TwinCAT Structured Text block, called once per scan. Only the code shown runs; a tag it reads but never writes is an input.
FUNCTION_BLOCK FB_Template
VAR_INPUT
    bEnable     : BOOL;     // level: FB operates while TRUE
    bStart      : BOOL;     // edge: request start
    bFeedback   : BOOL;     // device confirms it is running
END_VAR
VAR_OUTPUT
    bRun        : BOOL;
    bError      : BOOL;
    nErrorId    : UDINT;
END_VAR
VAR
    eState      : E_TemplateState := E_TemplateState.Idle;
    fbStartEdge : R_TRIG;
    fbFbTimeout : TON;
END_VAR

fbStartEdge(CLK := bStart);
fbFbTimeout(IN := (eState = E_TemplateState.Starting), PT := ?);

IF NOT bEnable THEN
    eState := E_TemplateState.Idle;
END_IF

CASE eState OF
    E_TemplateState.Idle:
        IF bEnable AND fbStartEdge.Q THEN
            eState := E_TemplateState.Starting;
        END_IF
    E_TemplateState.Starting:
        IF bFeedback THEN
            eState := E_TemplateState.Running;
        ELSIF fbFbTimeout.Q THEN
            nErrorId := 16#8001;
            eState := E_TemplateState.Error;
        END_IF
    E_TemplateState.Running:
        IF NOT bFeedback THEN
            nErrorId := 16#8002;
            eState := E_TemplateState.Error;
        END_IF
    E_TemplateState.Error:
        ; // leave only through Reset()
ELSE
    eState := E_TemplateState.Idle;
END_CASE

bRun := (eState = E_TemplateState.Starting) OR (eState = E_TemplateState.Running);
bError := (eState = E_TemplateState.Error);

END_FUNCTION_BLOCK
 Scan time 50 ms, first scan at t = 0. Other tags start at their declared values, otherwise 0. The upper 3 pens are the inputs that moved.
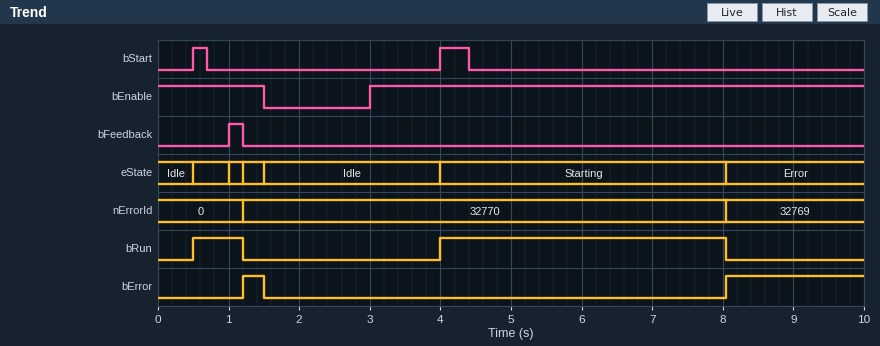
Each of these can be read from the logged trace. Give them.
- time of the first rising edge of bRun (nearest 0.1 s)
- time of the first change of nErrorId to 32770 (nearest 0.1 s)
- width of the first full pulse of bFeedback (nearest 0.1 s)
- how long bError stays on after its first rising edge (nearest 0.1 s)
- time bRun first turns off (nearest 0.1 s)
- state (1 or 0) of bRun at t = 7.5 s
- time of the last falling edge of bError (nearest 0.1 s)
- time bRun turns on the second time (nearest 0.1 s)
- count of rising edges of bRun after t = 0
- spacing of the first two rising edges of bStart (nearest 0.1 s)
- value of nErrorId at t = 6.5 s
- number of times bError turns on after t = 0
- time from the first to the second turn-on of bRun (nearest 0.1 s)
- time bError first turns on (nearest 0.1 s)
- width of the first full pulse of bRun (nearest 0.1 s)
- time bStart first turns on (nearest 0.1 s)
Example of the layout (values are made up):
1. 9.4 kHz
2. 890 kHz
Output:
1. 0.5 s
2. 1.2 s
3. 0.2 s
4. 0.3 s
5. 1.2 s
6. 1
7. 1.5 s
8. 4.0 s
9. 2
10. 3.5 s
11. 32770
12. 2
13. 3.5 s
14. 1.2 s
15. 0.7 s
16. 0.5 s
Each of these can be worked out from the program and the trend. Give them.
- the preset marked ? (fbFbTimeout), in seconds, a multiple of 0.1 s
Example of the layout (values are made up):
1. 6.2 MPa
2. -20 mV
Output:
1. 4.0 s
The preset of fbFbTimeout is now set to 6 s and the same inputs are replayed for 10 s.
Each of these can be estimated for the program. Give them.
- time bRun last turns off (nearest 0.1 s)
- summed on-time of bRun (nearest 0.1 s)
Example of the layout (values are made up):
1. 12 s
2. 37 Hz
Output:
1. 1.2 s
2. 6.7 s
